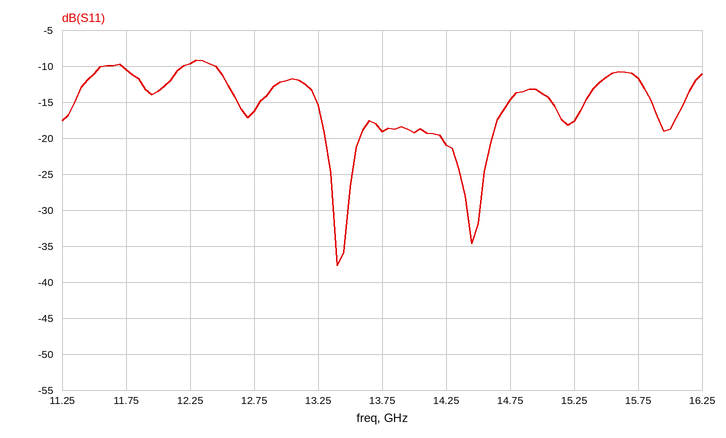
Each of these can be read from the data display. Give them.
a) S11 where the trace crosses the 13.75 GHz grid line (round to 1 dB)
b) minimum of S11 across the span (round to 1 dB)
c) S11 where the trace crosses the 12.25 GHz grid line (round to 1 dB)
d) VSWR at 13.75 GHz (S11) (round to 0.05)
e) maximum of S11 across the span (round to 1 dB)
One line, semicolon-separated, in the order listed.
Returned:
-19 dB; -38 dB; -10 dB; 1.25; -9 dB
